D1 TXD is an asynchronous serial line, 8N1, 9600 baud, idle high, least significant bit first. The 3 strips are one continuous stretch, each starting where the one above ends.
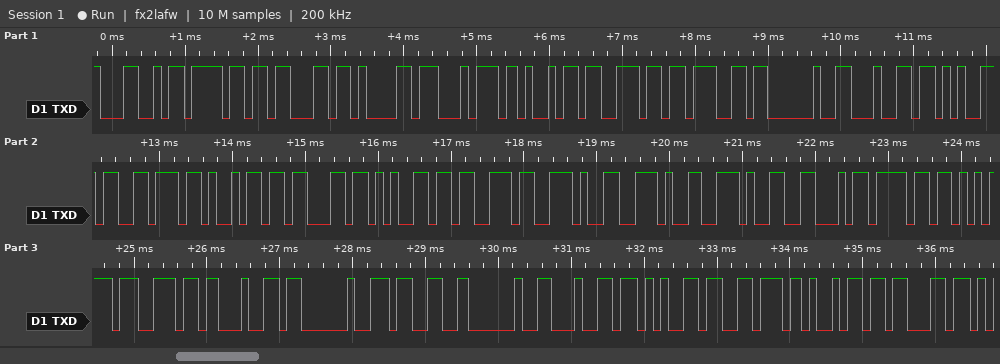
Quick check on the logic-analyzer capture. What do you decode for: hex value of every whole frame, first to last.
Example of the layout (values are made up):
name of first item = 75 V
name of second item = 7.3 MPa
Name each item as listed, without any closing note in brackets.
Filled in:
hex value of every whole frame, first to last = 4C 6F 63 61 74 69 6E 67 20 64 65 76 69 63 65 73 2E 2E 2E 46 6F 75 6E 64 20 33 20 64 65 76 69 63
